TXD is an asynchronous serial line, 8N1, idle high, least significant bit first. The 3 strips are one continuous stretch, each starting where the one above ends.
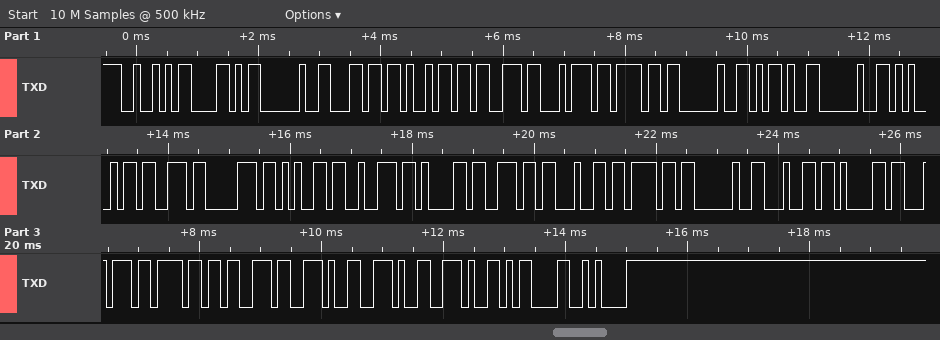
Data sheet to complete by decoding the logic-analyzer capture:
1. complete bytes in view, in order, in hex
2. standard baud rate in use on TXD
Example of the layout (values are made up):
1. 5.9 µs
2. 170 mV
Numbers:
1. 52 58 20 6C 69 73 74 6F 20 2D 20 45 73 70 65 72 61 6E 64 6F 20 64 61 74 6F 73 2E 2E 2E 0D 0A
2. 9600 baud
